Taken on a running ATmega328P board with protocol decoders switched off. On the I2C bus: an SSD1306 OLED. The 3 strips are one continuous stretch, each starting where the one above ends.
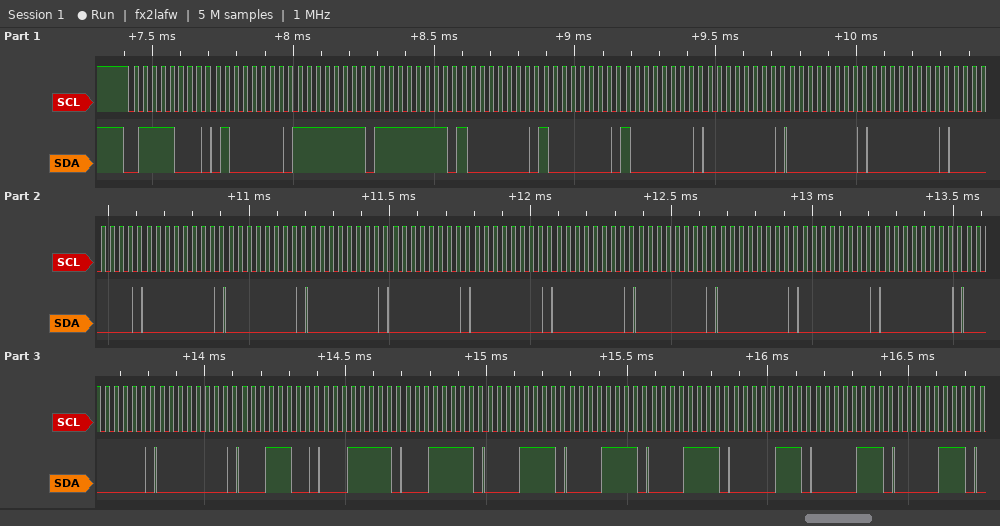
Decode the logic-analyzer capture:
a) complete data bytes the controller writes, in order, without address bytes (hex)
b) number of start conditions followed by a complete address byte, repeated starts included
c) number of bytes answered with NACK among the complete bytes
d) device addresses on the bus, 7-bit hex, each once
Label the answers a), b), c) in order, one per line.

a) 40 FF FF 80 80 80 00 00 00 00 00 00 00 00 00 00 00 00 00 00 00 00 1C 1F 1F 0F 0F 0F 07 07 07
b) 1
c) 0
d) 0x3C
